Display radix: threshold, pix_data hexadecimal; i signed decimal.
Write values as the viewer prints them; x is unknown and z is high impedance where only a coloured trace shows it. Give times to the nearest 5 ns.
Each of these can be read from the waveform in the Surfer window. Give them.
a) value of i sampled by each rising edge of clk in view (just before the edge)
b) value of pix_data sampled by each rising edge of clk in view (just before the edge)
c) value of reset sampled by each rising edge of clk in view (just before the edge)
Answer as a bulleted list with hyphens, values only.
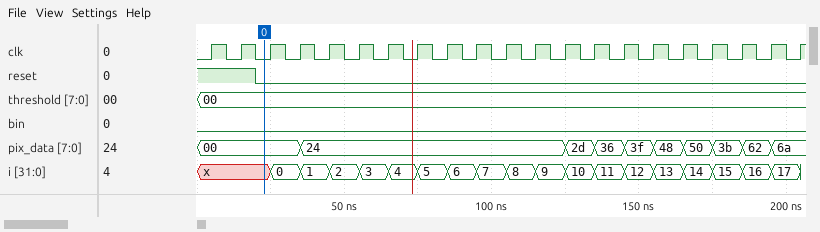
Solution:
- x, x, x, 0, 1, 2, 3, 4, 5, 6, 7, 8, 9, 10, 11, 12, 13, 14, 15, 16, 17
- 00, 00, 00, 00, 24, 24, 24, 24, 24, 24, 24, 24, 24, 2d, 36, 3f, 48, 50, 3b, 62, 6a
- 1 1 0 0 0 0 0 0 0 0 0 0 0 0 0 0 0 0 0 0 0
